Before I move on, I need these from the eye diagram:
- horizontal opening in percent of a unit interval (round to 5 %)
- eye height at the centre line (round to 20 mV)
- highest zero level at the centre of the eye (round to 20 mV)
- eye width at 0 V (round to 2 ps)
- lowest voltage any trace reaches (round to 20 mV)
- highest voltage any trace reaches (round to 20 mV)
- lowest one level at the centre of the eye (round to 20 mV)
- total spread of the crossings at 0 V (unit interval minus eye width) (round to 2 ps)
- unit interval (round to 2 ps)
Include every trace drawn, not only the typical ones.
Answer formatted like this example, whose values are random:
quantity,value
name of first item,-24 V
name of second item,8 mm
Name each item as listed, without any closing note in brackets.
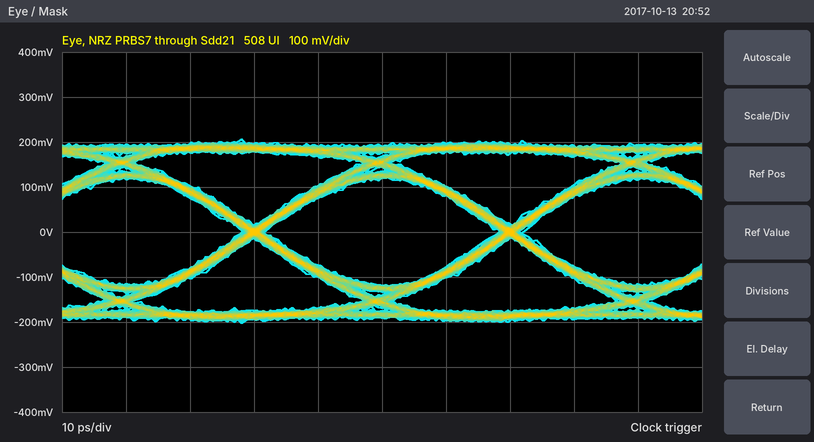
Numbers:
quantity,value
horizontal opening in percent of a unit interval,90 %
eye height at the centre line,240 mV
highest zero level at the centre of the eye,-120 mV
eye width at 0 V,36 ps
lowest voltage any trace reaches,-200 mV
highest voltage any trace reaches,200 mV
lowest one level at the centre of the eye,120 mV
total spread of the crossings at 0 V (unit interval minus eye width),4 ps
unit interval,40 ps
